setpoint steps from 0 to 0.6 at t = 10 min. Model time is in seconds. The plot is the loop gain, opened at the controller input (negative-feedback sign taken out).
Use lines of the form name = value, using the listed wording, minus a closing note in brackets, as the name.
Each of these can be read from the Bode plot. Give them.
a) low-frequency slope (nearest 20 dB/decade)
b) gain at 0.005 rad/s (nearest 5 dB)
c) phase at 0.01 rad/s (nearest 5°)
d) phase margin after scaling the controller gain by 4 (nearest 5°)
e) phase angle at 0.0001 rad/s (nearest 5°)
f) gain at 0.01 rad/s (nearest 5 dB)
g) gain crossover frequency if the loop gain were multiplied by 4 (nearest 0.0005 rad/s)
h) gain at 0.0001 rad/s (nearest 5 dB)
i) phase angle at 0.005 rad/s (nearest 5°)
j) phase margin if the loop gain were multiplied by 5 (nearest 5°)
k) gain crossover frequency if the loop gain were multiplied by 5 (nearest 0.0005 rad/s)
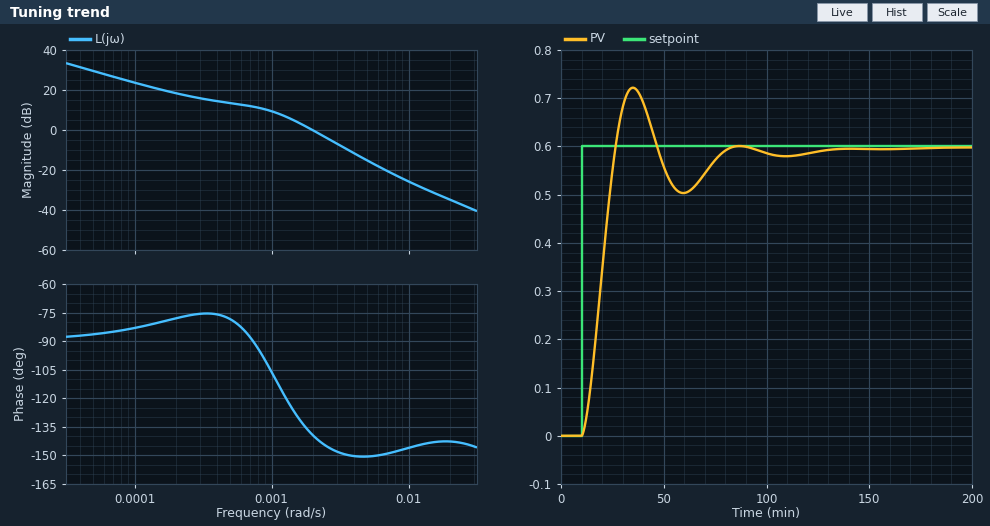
low-frequency slope = -20 dB/decade
gain at 0.005 rad/s = -15 dB
phase at 0.01 rad/s = -145°
phase margin after scaling the controller gain by 4 = 30°
phase angle at 0.0001 rad/s = -85°
gain at 0.01 rad/s = -25 dB
gain crossover frequency if the loop gain were multiplied by 4 = 0.0040 rad/s
gain at 0.0001 rad/s = 25 dB
phase angle at 0.005 rad/s = -150°
phase margin if the loop gain were multiplied by 5 = 30°
gain crossover frequency if the loop gain were multiplied by 5 = 0.0045 rad/s
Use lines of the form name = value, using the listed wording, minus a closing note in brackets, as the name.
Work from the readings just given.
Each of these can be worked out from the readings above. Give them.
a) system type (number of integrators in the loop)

system type = 1
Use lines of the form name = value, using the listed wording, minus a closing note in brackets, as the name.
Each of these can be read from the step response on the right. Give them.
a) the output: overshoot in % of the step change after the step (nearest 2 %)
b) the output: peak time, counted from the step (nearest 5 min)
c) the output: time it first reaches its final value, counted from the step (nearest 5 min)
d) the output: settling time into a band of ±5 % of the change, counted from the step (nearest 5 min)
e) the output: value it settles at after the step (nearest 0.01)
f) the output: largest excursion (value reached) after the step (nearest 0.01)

the output: overshoot in % of the step change after the step = 20 %
the output: peak time, counted from the step = 25 min
the output: time it first reaches its final value, counted from the step = 15 min
the output: settling time into a band of ±5 % of the change, counted from the step = 65 min
the output: value it settles at after the step = 0.60
the output: largest excursion (value reached) after the step = 0.72
